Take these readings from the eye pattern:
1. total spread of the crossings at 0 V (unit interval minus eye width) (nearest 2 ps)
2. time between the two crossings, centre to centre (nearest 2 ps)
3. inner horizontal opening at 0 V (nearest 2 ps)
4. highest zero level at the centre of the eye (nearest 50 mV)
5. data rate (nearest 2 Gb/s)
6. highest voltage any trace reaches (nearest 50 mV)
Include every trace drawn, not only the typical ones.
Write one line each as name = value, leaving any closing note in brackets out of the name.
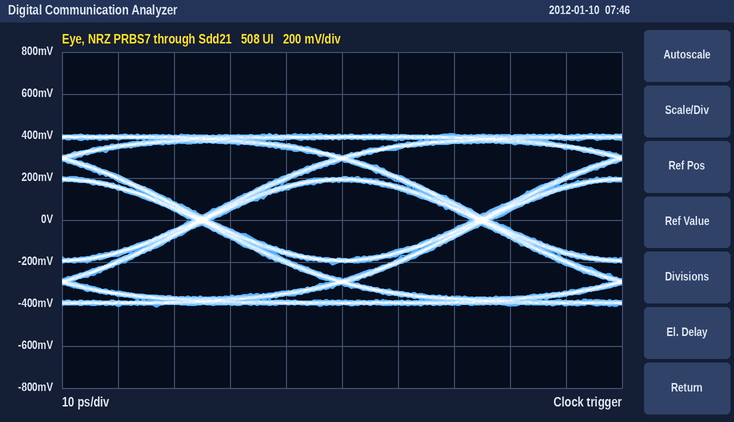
total spread of the crossings at 0 V (unit interval minus eye width) = 4 ps
time between the two crossings, centre to centre = 50 ps
inner horizontal opening at 0 V = 46 ps
highest zero level at the centre of the eye = -200 mV
data rate = 20 Gb/s
highest voltage any trace reaches = 400 mV
